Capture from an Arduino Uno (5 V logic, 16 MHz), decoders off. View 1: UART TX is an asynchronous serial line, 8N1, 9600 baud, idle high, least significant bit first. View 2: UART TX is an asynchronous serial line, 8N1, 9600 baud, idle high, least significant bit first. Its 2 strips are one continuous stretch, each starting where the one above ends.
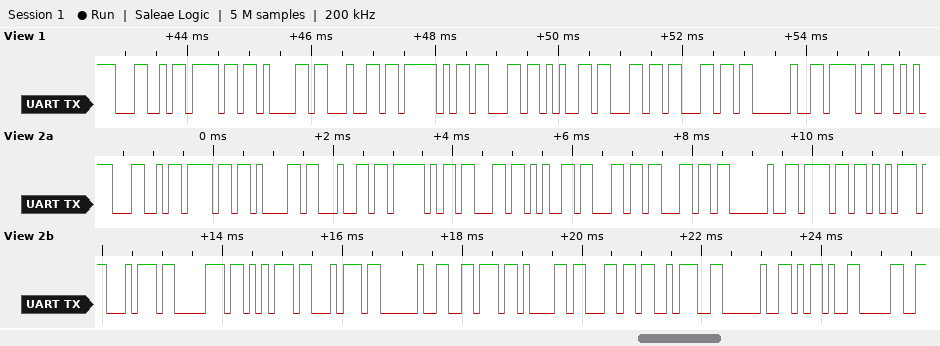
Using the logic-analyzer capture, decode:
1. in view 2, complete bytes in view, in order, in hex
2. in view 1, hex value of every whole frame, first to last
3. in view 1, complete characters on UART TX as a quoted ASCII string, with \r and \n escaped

0x4C 0x6F 0x61 0x64 0x5F 0x63 0x65 0x6C 0x6C 0x20 0x6F 0x75 0x74 0x70 0x75 0x74 0x20 0x76 0x61 0x6C 0x3A 0x20 0x2D 0x30
4C 6F 61 64 5F 63 65 6C 6C 20 6F
"Load_cell o"
